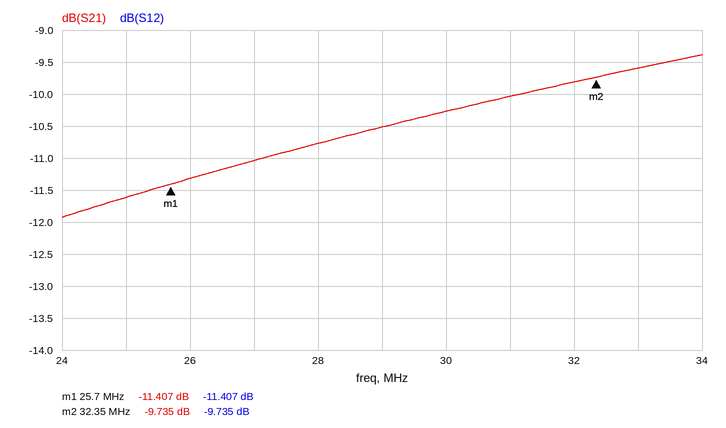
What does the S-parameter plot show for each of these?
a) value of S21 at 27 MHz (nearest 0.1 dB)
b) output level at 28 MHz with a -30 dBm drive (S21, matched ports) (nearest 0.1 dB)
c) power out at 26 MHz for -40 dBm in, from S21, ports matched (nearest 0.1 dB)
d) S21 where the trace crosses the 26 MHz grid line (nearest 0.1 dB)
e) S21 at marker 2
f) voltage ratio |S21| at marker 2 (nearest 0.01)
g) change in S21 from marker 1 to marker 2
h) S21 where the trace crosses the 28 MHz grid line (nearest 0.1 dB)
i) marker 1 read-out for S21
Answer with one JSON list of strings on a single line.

["-11.0 dB", "-40.8 dBm", "-51.3 dBm", "-11.3 dB", "-9.735 dB", "0.33", "1.672 dB", "-10.8 dB", "-11.407 dB"]
